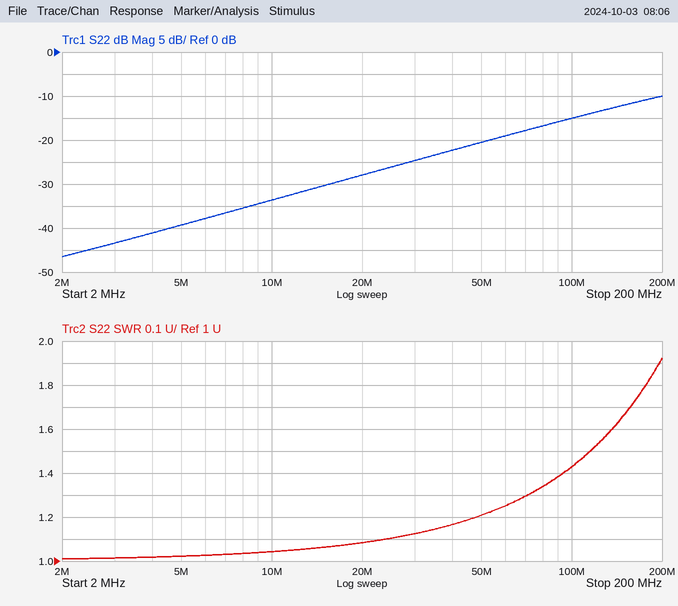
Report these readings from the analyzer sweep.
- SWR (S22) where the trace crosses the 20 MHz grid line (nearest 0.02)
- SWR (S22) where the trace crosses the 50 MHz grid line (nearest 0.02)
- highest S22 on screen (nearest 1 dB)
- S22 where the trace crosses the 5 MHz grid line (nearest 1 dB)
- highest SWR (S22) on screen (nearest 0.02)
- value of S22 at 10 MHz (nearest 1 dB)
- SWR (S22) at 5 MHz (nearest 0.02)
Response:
1.08
1.20
-10 dB
-39 dB
1.92
-34 dB
1.02
